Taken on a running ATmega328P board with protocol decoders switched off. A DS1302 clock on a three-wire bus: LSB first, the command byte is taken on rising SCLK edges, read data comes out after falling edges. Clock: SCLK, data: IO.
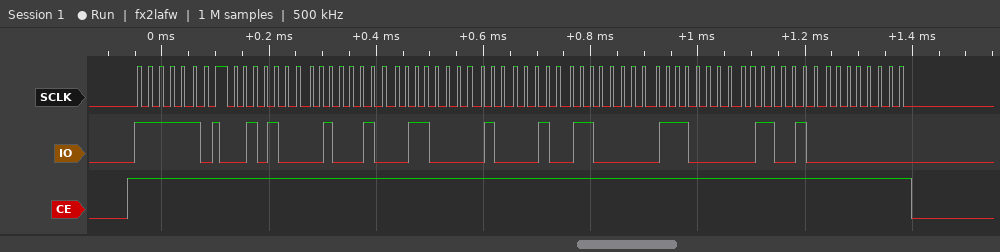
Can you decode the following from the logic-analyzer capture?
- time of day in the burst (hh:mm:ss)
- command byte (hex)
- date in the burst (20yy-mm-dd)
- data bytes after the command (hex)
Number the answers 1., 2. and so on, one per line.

1. 06:22:14
2. 0xBF
3. 2026-03-21
4. 14 22 06 21 03 07 26 00
